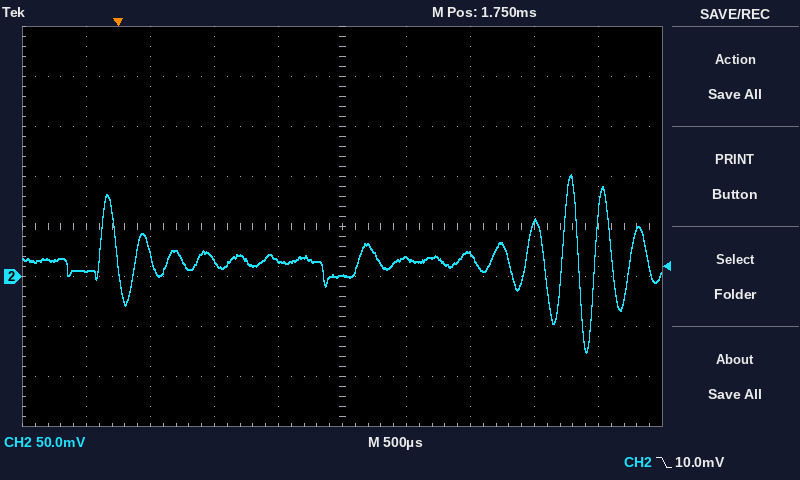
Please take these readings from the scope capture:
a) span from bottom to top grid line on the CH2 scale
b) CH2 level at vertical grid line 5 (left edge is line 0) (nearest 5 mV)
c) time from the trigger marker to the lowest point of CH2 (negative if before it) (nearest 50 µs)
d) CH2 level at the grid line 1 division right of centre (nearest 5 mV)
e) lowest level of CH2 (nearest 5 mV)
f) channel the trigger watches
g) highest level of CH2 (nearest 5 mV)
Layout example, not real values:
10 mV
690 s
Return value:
400 mV
0 mV
+3.65 ms
20 mV
-75 mV
CH2
100 mV
